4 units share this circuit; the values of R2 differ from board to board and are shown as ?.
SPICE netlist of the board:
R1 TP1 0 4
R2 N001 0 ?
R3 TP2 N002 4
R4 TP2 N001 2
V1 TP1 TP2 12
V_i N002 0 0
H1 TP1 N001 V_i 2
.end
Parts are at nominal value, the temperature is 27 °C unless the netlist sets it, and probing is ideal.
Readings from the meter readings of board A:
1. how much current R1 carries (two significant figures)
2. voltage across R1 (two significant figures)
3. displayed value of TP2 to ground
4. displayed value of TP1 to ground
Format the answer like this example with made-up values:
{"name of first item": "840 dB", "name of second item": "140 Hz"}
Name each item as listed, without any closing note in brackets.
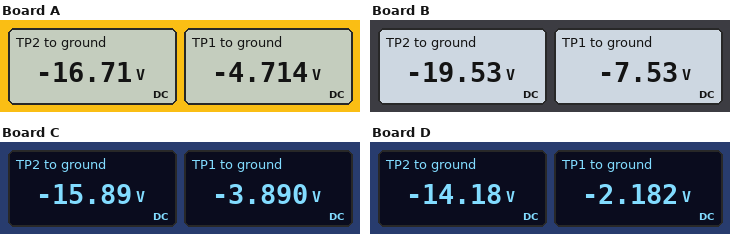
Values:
{"how much current R1 carries": "1.2 A", "voltage across R1": "4.7 V", "displayed value of TP2 to ground": "-16.71 V", "displayed value of TP1 to ground": "-4.714 V"}
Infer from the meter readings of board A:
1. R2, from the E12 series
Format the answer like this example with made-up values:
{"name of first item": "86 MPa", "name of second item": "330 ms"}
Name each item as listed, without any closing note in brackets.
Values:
{"R2, from the E12 series": "0.68 Ω"}
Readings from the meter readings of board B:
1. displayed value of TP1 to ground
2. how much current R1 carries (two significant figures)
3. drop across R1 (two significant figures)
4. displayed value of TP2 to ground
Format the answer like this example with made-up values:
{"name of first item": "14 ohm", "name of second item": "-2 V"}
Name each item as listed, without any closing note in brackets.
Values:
{"displayed value of TP1 to ground": "-7.53 V", "how much current R1 carries": "1.9 A", "drop across R1": "7.5 V", "displayed value of TP2 to ground": "-19.53 V"}
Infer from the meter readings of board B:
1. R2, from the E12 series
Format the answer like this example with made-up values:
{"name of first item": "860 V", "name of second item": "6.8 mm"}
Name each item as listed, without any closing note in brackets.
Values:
{"R2, from the E12 series": "0.33 Ω"}
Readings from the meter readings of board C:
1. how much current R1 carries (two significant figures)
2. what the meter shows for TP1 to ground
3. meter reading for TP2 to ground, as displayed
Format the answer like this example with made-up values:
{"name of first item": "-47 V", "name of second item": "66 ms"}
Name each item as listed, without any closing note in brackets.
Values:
{"how much current R1 carries": "970 mA", "what the meter shows for TP1 to ground": "-3.890 V", "meter reading for TP2 to ground, as displayed": "-15.89 V"}
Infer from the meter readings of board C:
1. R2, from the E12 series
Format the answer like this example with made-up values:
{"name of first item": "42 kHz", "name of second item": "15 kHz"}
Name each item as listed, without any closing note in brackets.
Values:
{"R2, from the E12 series": "0.82 Ω"}
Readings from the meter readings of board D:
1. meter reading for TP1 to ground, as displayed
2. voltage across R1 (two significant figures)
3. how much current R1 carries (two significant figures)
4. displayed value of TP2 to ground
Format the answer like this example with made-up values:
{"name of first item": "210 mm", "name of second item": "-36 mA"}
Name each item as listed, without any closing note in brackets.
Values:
{"meter reading for TP1 to ground, as displayed": "-2.182 V", "voltage across R1": "2.2 V", "how much current R1 carries": "550 mA", "displayed value of TP2 to ground": "-14.18 V"}
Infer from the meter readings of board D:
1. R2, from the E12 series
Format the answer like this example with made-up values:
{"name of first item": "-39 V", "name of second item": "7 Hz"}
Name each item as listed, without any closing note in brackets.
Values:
{"R2, from the E12 series": "1.2 Ω"}
